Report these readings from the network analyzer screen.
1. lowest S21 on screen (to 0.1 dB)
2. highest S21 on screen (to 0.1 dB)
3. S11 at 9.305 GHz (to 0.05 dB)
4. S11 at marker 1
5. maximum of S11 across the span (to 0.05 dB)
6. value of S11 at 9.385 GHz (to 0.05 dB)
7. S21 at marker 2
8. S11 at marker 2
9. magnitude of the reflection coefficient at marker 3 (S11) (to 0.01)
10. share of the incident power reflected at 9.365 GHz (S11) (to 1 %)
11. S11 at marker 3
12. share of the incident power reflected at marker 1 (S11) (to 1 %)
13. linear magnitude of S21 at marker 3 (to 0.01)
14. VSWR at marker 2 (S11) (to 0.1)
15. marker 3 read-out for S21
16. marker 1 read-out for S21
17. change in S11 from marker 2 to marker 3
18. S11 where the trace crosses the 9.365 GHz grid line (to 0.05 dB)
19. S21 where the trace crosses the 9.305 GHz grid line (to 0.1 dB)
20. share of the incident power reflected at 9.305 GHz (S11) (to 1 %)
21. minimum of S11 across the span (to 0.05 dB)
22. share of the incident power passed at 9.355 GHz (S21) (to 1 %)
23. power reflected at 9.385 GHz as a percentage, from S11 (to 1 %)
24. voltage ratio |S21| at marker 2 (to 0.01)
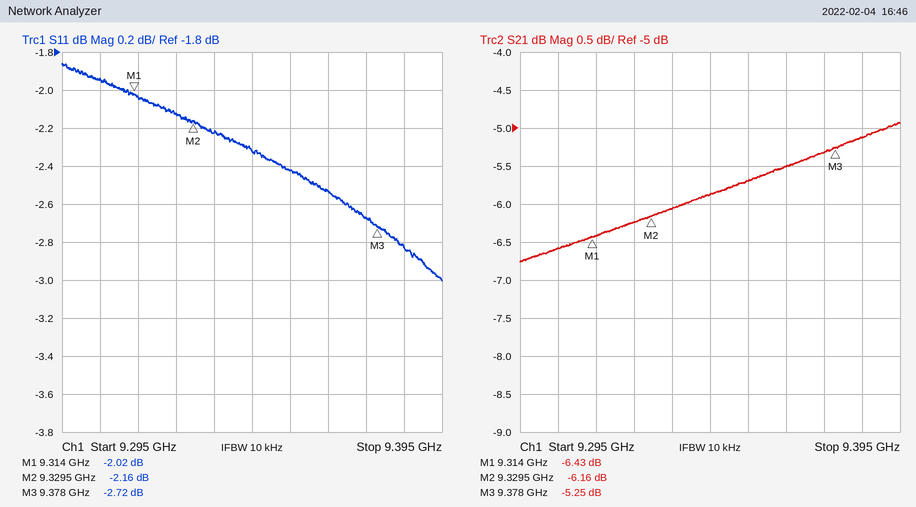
-6.8 dB
-4.9 dB
-1.95 dB
-2.02 dB
-1.85 dB
-2.85 dB
-6.16 dB
-2.16 dB
0.73
56 %
-2.72 dB
63 %
0.55
8.1
-5.25 dB
-6.43 dB
-0.56 dB
-2.55 dB
-6.6 dB
64 %
-3.00 dB
27 %
52 %
0.49
